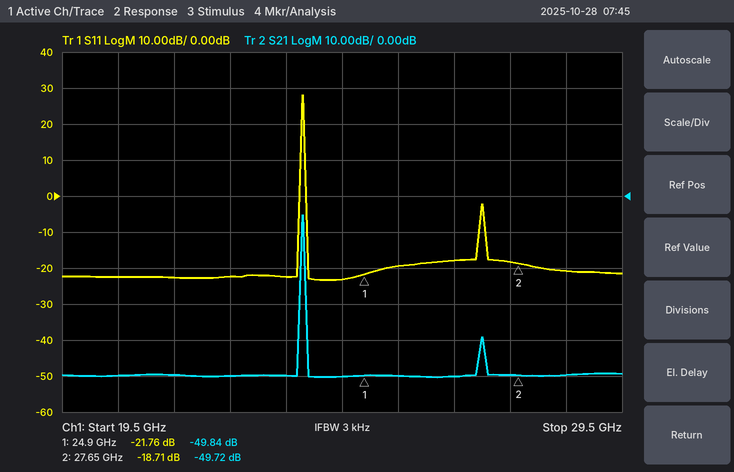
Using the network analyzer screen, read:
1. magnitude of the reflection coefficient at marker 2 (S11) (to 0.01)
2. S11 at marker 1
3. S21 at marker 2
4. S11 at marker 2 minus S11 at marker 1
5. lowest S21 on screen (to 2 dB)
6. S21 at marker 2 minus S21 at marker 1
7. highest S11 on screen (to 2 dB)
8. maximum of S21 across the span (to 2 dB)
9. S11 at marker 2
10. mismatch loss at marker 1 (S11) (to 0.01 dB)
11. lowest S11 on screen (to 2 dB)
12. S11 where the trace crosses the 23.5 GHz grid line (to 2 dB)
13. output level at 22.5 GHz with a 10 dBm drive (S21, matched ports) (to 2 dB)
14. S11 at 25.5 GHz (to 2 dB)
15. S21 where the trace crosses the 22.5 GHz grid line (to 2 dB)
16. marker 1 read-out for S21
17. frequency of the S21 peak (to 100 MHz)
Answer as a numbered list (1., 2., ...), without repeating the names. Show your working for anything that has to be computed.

1. 10^(-18.71/20) ≈ 0.12
2. -21.76 dB
3. -49.72 dB
4. -18.71 − (-21.76) = 3.05 dB
5. -50 dB
6. -49.72 − (-49.84) = 0.12 dB
7. 28 dB
8. -6 dB
9. -18.71 dB
10. −10 log10(1 − 10^(-21.76/10)) ≈ 0.03 dB
11. -24 dB
12. -22 dB
13. 10 dBm + (-50 dB) = -40 dBm
14. -20 dB
15. -50 dB
16. -49.84 dB
17. 23.8 GHz
